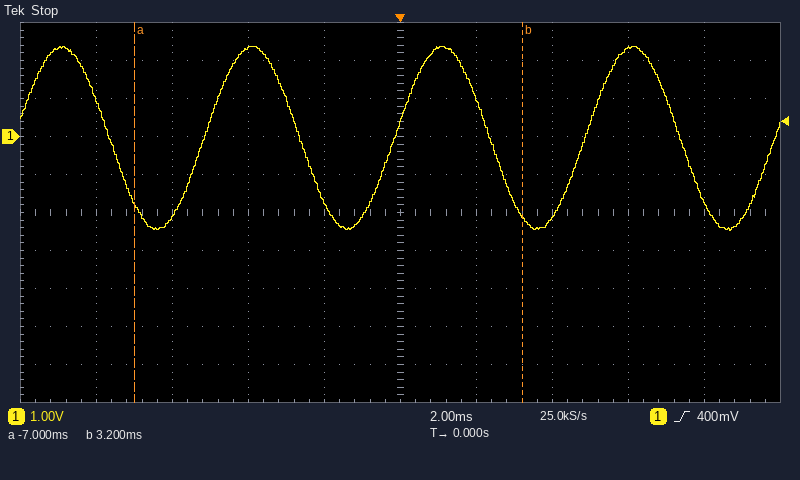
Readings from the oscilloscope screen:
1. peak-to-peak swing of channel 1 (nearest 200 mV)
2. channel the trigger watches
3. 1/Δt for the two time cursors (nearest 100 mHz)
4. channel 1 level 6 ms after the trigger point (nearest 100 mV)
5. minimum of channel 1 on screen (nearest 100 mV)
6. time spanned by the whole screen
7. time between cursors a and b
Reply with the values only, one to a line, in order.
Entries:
4.8 V
channel 1
98.0 Hz
2.3 V
-2.5 V
20 ms
10.2 ms
